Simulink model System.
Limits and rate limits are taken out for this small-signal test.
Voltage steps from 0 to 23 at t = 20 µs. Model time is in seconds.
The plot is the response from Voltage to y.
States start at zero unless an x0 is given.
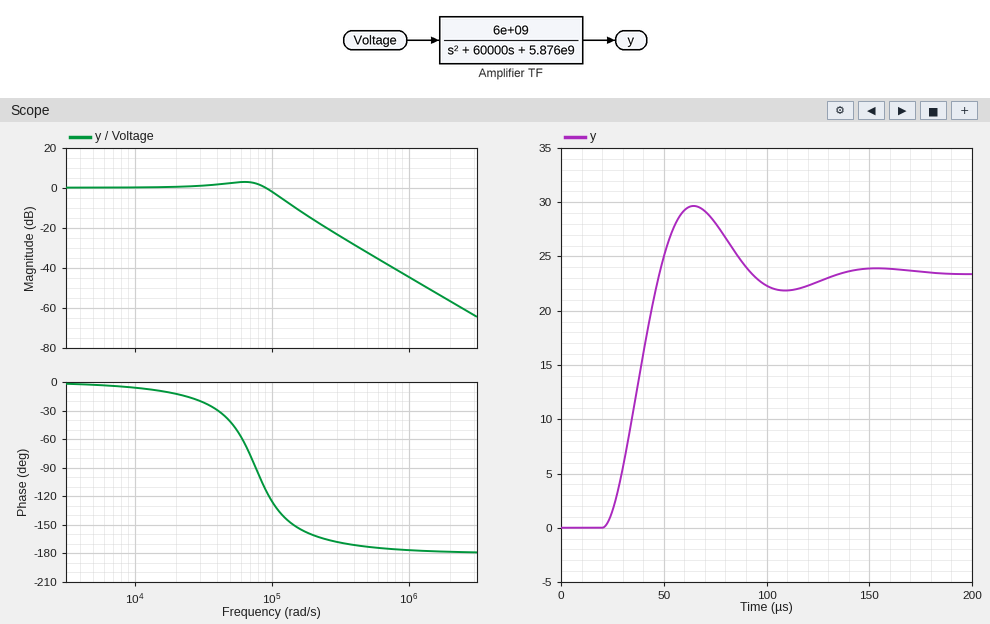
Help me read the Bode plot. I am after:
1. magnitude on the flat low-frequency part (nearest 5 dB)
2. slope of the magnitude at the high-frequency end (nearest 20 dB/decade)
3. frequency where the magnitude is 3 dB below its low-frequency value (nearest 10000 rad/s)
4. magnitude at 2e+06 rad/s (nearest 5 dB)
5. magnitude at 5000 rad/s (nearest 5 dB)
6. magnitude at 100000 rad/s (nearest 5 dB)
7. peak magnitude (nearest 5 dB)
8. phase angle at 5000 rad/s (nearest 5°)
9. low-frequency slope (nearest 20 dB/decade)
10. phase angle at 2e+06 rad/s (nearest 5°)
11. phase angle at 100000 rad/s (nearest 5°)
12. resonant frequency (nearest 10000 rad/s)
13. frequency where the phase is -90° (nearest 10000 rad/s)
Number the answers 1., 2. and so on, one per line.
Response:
1. 0 dB
2. -40 dB/decade
3. 110000 rad/s
4. -55 dB
5. 0 dB
6. 0 dB
7. 5 dB
8. -5°
9. 0 dB/decade
10. -180°
11. -125°
12. 60000 rad/s
13. 80000 rad/s
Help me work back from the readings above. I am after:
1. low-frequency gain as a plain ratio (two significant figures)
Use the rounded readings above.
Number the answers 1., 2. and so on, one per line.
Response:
1. 1.0
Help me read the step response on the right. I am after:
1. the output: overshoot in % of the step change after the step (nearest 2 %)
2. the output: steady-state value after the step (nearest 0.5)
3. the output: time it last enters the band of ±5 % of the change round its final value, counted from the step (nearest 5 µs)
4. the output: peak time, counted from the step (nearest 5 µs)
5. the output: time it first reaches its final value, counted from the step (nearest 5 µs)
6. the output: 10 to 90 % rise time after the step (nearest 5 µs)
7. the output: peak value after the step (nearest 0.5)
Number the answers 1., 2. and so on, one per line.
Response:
1. 26 %
2. 23.5
3. 100 µs
4. 45 µs
5. 30 µs
6. 20 µs
7. 29.5
